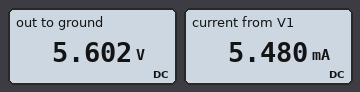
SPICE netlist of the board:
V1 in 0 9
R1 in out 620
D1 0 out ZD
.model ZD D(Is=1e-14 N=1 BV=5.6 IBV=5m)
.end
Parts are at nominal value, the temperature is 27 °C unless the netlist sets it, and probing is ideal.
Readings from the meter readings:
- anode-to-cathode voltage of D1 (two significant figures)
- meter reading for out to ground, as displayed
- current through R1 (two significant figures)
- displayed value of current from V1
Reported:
-5.6 V
5.602 V
5.5 mA
5.480 mA
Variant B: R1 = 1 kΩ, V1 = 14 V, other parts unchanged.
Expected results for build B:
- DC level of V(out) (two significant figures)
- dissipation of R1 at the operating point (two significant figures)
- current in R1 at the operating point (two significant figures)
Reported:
5.6 V
70 mW
8.4 mA
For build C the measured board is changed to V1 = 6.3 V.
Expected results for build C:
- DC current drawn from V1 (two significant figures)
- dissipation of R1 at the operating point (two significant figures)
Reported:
1.2 mA
880 µW
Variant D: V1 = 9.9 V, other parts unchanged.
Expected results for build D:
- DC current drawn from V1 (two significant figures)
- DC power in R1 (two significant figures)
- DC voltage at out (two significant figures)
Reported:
6.9 mA
30 mW
5.6 V
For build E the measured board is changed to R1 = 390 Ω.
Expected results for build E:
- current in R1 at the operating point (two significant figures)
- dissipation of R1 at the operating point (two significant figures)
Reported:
8.7 mA
29 mW
